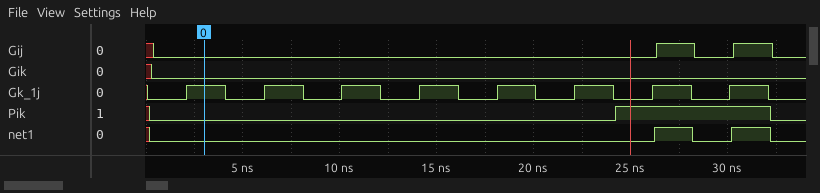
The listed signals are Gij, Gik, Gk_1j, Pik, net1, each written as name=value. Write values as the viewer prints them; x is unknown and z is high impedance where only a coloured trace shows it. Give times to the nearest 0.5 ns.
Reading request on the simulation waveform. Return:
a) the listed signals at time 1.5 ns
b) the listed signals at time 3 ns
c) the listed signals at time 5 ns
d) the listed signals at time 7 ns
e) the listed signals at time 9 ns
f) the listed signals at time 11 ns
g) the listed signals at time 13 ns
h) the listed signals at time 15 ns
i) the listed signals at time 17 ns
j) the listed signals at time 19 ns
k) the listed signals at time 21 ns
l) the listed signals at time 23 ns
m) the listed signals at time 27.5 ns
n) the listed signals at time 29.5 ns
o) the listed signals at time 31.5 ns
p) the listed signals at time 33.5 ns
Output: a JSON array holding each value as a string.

["Gij=0, Gik=0, Gk_1j=0, Pik=0, net1=0", "Gij=0, Gik=0, Gk_1j=1, Pik=0, net1=0", "Gij=0, Gik=0, Gk_1j=0, Pik=0, net1=0", "Gij=0, Gik=0, Gk_1j=1, Pik=0, net1=0", "Gij=0, Gik=0, Gk_1j=0, Pik=0, net1=0", "Gij=0, Gik=0, Gk_1j=1, Pik=0, net1=0", "Gij=0, Gik=0, Gk_1j=0, Pik=0, net1=0", "Gij=0, Gik=0, Gk_1j=1, Pik=0, net1=0", "Gij=0, Gik=0, Gk_1j=0, Pik=0, net1=0", "Gij=0, Gik=0, Gk_1j=1, Pik=0, net1=0", "Gij=0, Gik=0, Gk_1j=0, Pik=0, net1=0", "Gij=0, Gik=0, Gk_1j=1, Pik=0, net1=0", "Gij=1, Gik=0, Gk_1j=1, Pik=1, net1=1", "Gij=0, Gik=0, Gk_1j=0, Pik=1, net1=0", "Gij=1, Gik=0, Gk_1j=1, Pik=1, net1=1", "Gij=0, Gik=0, Gk_1j=0, Pik=0, net1=0"]
